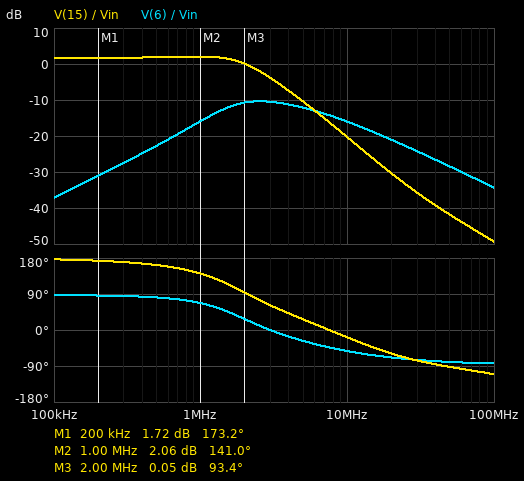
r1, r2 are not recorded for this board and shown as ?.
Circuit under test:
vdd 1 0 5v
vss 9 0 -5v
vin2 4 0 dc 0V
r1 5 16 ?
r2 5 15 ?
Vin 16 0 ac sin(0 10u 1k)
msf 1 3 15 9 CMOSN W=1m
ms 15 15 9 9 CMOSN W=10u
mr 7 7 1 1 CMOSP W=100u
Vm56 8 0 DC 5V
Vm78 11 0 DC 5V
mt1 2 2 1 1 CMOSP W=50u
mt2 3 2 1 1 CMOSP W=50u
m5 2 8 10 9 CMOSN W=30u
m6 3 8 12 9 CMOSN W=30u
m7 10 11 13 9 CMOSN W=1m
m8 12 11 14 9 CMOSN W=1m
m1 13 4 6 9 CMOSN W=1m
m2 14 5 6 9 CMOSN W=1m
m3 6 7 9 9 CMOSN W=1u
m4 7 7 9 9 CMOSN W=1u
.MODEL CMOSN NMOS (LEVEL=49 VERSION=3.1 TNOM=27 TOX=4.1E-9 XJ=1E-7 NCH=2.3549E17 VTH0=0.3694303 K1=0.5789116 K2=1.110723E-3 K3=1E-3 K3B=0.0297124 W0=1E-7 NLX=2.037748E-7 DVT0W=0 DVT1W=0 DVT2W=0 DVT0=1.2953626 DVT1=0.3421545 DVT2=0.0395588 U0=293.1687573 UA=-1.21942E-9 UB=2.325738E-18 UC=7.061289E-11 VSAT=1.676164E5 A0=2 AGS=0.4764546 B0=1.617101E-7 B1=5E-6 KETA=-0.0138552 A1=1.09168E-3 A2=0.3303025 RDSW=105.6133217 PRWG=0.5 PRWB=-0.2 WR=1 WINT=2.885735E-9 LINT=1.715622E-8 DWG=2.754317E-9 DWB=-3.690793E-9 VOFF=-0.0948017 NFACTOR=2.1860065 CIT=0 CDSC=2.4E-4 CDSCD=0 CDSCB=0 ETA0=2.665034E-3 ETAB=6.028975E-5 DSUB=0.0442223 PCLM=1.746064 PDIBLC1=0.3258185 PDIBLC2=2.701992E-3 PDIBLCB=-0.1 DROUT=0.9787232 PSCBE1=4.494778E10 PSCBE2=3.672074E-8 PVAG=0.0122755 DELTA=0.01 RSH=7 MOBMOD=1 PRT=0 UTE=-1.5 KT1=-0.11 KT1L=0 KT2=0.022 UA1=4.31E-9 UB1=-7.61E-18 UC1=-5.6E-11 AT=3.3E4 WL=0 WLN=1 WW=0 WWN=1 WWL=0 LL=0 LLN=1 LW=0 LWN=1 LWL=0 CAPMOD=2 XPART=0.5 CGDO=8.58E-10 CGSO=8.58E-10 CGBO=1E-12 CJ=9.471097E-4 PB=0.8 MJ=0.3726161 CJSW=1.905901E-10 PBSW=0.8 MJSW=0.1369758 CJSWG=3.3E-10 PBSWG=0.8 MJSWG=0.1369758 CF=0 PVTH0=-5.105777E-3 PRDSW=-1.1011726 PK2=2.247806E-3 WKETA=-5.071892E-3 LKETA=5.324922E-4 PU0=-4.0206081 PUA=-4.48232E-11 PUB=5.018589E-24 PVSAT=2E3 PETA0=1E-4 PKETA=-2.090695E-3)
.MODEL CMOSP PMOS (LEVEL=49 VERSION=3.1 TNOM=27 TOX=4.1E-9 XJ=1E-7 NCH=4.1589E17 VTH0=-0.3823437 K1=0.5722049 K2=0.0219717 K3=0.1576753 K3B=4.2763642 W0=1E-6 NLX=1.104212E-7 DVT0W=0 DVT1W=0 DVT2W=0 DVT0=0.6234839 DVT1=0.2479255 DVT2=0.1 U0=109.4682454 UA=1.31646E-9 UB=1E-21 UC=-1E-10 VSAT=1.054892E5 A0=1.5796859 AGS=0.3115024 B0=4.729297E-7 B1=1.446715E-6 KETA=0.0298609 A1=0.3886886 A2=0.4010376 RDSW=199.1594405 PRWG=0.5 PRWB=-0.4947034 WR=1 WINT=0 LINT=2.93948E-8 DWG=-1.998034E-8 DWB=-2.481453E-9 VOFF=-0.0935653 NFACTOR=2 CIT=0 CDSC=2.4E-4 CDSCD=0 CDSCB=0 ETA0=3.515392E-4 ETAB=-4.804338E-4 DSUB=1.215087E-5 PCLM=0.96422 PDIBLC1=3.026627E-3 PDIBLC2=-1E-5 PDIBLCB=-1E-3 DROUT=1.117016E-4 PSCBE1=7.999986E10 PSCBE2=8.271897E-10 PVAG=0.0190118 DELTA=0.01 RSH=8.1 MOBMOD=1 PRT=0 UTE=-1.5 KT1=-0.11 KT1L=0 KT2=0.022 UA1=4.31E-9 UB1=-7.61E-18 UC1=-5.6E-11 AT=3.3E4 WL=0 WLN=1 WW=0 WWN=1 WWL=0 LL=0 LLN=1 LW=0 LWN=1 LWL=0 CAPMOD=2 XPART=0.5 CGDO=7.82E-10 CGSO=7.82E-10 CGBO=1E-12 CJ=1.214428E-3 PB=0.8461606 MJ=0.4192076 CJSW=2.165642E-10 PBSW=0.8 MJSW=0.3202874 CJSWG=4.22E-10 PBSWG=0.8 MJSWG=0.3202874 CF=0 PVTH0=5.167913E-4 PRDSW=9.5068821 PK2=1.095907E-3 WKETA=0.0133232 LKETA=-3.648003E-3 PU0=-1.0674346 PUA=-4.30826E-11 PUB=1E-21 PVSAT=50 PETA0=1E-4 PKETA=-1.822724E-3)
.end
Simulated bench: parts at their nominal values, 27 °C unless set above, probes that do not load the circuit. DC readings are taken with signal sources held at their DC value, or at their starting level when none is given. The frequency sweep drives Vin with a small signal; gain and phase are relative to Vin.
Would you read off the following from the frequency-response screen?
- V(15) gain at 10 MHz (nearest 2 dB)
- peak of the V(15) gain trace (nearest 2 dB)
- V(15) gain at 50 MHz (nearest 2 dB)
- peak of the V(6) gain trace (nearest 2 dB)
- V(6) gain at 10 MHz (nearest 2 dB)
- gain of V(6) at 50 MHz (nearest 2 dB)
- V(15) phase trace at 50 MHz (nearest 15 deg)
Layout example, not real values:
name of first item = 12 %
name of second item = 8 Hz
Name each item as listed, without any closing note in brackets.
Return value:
V(15) gain at 10 MHz = -20 dB
peak of the V(15) gain trace = 2 dB
V(15) gain at 50 MHz = -42 dB
peak of the V(6) gain trace = -10 dB
V(6) gain at 10 MHz = -16 dB
gain of V(6) at 50 MHz = -28 dB
V(15) phase trace at 50 MHz = -90 deg
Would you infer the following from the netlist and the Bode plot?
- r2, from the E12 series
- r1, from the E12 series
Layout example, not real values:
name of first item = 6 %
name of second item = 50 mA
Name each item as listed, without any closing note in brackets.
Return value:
r2, from the E12 series = 3.3 kΩ
r1, from the E12 series = 2.7 kΩ
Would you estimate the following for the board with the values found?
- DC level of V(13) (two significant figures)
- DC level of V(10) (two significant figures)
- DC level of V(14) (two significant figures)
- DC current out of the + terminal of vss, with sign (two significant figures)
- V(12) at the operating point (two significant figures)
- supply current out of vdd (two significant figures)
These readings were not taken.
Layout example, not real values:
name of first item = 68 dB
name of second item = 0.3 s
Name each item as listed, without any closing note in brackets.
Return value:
DC level of V(13) = 3.1 V
DC level of V(10) = 3.1 V
DC level of V(14) = 1.5 V
DC current out of the + terminal of vss, with sign = -3.0 mA
V(12) at the operating point = 1.5 V
supply current out of vdd = 3.0 mA
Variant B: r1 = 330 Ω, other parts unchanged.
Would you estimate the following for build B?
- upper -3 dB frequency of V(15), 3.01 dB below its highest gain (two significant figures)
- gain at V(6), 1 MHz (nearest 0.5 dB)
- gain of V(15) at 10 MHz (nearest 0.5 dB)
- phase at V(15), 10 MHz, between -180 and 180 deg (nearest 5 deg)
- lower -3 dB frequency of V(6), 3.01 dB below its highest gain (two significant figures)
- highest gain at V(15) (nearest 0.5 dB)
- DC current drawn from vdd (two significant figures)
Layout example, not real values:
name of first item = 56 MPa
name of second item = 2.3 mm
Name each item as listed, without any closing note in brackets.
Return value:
upper -3 dB frequency of V(15), 3.01 dB below its highest gain = 410 kHz
gain at V(6), 1 MHz = -7.5 dB
gain of V(15) at 10 MHz = -12.5 dB
phase at V(15), 10 MHz, between -180 and 180 deg = 20 deg
lower -3 dB frequency of V(6), 3.01 dB below its highest gain = 350 kHz
highest gain at V(15) = 19.5 dB
DC current drawn from vdd = 3.1 mA
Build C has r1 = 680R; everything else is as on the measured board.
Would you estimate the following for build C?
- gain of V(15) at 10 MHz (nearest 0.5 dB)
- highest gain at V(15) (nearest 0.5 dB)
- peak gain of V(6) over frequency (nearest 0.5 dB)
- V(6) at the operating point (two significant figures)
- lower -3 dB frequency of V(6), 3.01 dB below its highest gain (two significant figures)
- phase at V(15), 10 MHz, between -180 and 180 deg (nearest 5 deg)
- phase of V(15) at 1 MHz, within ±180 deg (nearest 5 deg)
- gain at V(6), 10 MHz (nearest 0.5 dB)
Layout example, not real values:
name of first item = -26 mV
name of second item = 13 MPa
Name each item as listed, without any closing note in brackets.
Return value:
gain of V(15) at 10 MHz = -13.5 dB
highest gain at V(15) = 13.5 dB
peak gain of V(6) over frequency = -8.0 dB
V(6) at the operating point = -1.1 V
lower -3 dB frequency of V(6), 3.01 dB below its highest gain = 610 kHz
phase at V(15), 10 MHz, between -180 and 180 deg = 10 deg
phase of V(15) at 1 MHz, within ±180 deg = 105 deg
gain at V(6), 10 MHz = -9.5 dB
